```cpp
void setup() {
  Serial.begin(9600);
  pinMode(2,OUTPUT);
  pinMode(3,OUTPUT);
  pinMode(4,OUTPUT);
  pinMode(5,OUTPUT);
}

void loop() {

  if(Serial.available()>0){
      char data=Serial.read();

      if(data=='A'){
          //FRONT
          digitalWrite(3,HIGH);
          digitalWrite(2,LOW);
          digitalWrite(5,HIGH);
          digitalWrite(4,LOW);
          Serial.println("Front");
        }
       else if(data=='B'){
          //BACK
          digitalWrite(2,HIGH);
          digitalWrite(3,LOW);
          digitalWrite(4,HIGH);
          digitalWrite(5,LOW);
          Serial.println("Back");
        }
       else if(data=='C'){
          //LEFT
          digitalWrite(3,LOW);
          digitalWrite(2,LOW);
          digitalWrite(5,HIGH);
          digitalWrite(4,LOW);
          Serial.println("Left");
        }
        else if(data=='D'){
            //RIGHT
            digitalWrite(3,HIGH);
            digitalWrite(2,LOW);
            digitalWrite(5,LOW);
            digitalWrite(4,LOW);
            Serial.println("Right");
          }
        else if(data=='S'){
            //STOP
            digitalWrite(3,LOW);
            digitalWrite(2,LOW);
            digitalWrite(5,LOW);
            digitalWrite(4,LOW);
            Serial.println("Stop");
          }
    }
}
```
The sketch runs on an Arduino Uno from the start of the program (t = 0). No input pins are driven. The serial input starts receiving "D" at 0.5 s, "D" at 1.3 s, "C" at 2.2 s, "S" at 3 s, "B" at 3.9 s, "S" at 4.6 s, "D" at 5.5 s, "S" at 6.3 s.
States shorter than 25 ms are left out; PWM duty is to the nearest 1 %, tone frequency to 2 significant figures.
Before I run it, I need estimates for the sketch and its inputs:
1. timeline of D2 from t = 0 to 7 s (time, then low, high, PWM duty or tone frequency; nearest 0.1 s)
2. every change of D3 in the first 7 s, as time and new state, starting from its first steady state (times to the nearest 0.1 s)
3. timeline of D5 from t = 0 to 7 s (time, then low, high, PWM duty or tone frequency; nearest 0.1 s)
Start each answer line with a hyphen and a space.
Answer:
- 0 s low; 3.9 s high; 4.6 s low
- 0 s low; 0.5 s high; 2.2 s low; 5.5 s high; 6.3 s low
- 0 s low; 2.2 s high; 3 s low
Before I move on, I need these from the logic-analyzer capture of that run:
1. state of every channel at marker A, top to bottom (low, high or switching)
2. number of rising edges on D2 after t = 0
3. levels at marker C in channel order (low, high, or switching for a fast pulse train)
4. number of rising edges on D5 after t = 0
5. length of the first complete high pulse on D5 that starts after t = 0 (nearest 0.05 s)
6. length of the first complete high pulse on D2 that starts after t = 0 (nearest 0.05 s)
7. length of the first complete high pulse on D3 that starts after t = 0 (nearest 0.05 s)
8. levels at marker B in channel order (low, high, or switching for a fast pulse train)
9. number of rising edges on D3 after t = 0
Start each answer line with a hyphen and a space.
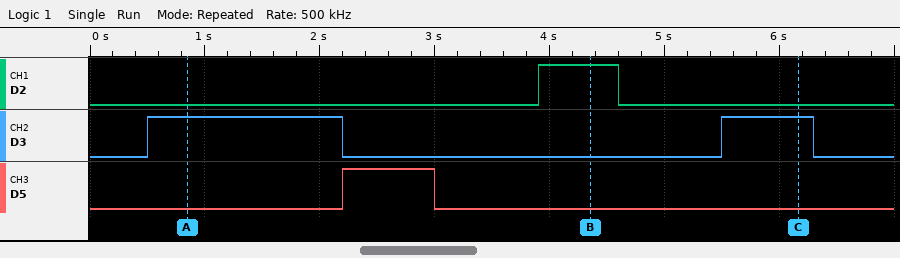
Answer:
- D2 low, D3 high, D5 low
- 1
- D2 low, D3 high, D5 low
- 1
- 0.80 s
- 0.70 s
- 1.70 s
- D2 high, D3 low, D5 low
- 2
